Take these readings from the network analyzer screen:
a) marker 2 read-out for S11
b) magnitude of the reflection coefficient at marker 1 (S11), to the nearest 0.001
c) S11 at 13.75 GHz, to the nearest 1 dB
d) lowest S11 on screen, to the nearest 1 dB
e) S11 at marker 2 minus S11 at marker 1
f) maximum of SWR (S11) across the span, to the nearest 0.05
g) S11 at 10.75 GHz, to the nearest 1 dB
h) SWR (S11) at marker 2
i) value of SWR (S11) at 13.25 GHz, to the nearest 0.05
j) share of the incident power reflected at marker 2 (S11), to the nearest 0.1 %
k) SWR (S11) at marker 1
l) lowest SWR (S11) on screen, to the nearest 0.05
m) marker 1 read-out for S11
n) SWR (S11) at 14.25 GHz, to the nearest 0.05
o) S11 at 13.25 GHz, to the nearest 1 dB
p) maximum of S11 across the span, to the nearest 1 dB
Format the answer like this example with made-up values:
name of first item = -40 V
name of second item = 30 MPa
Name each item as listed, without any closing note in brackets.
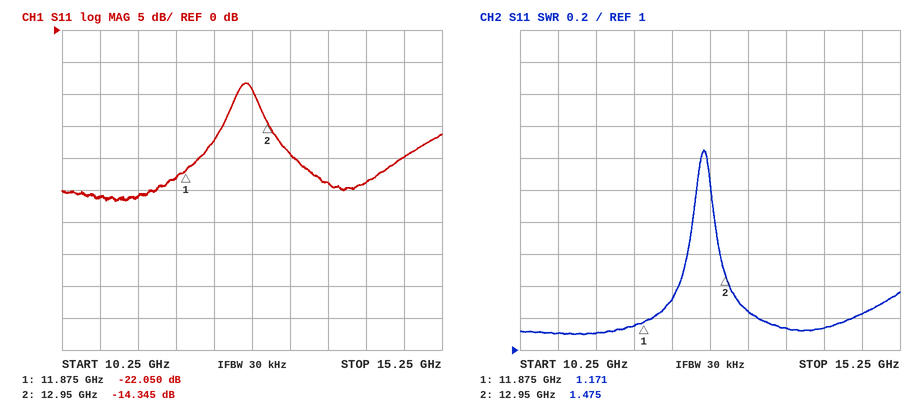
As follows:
marker 2 read-out for S11 = -14.345 dB
magnitude of the reflection coefficient at marker 1 (S11), to the nearest 0.001 = 0.079
S11 at 13.75 GHz, to the nearest 1 dB = -24 dB
lowest S11 on screen, to the nearest 1 dB = -27 dB
S11 at marker 2 minus S11 at marker 1 = 7.705 dB
maximum of SWR (S11) across the span, to the nearest 0.05 = 2.25
S11 at 10.75 GHz, to the nearest 1 dB = -26 dB
SWR (S11) at marker 2 = 1.475
value of SWR (S11) at 13.25 GHz, to the nearest 0.05 = 1.25
share of the incident power reflected at marker 2 (S11), to the nearest 0.1 % = 3.7 %
SWR (S11) at marker 1 = 1.171
lowest SWR (S11) on screen, to the nearest 0.05 = 1.10
marker 1 read-out for S11 = -22.050 dB
SWR (S11) at 14.25 GHz, to the nearest 0.05 = 1.15
S11 at 13.25 GHz, to the nearest 1 dB = -19 dB
maximum of S11 across the span, to the nearest 1 dB = -8 dB
